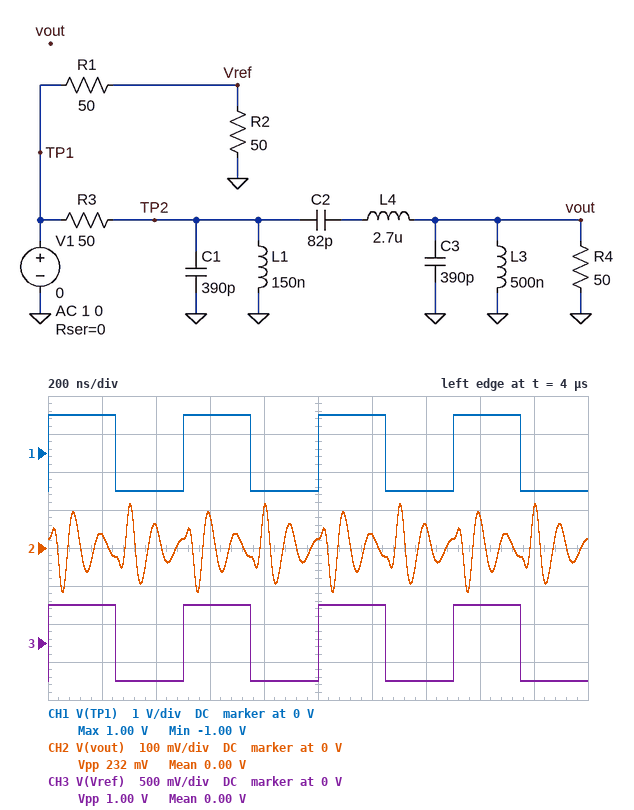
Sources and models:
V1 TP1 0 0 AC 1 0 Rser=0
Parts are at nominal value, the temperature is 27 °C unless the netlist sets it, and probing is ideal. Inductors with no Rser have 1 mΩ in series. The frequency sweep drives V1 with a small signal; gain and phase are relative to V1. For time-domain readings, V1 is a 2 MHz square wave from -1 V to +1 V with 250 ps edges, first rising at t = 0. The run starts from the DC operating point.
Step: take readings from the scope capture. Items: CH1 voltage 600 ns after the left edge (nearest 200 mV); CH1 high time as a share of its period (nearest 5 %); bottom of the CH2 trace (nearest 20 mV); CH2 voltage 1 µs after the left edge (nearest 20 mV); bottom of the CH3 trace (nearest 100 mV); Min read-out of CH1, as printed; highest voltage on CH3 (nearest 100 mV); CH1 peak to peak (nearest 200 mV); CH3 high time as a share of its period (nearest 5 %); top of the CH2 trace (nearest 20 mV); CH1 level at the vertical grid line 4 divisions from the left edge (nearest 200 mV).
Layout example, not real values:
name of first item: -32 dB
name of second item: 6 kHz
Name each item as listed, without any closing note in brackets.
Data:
CH1 voltage 600 ns after the left edge: 1.0 V
CH1 high time as a share of its period: 50 %
bottom of the CH2 trace: -120 mV
CH2 voltage 1 µs after the left edge: 20 mV
bottom of the CH3 trace: -500 mV
Min read-out of CH1, as printed: -1.00 V
highest voltage on CH3: 500 mV
CH1 peak to peak: 2.0 V
CH3 high time as a share of its period: 50 %
top of the CH2 trace: 120 mV
CH1 level at the vertical grid line 4 divisions from the left edge: -1.0 V
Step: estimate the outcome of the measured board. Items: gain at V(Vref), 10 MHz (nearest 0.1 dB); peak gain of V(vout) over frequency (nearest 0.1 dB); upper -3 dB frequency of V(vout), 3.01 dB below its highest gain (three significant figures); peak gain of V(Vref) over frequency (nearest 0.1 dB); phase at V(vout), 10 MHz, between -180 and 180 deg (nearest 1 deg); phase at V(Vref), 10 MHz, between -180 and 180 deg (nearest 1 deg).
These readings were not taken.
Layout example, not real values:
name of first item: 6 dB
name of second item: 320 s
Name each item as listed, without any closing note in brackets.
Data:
gain at V(Vref), 10 MHz: -6.0 dB
peak gain of V(vout) over frequency: -12.5 dB
upper -3 dB frequency of V(vout), 3.01 dB below its highest gain: 14.3 MHz
peak gain of V(Vref) over frequency: -6.0 dB
phase at V(vout), 10 MHz, between -180 and 180 deg: 92 deg
phase at V(Vref), 10 MHz, between -180 and 180 deg: 0 deg
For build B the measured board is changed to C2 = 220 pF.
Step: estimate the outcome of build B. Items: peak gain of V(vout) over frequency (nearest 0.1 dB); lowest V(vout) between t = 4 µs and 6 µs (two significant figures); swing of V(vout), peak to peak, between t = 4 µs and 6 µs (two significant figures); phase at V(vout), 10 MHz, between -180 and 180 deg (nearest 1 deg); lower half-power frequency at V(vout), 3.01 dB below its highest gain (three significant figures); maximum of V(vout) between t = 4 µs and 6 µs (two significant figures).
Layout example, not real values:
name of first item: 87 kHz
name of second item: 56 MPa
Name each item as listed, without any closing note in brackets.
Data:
peak gain of V(vout) over frequency: -12.1 dB
lowest V(vout) between t = 4 µs and 6 µs: -130 mV
swing of V(vout), peak to peak, between t = 4 µs and 6 µs: 260 mV
phase at V(vout), 10 MHz, between -180 and 180 deg: 27 deg
lower half-power frequency at V(vout), 3.01 dB below its highest gain: 5.60 MHz
maximum of V(vout) between t = 4 µs and 6 µs: 130 mV
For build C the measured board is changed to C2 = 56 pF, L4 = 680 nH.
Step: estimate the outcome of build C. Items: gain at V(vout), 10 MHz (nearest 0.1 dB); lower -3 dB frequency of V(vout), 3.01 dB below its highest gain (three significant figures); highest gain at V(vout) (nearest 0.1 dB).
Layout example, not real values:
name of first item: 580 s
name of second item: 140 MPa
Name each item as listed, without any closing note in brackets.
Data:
gain at V(vout), 10 MHz: -25.8 dB
lower -3 dB frequency of V(vout), 3.01 dB below its highest gain: 28.2 MHz
highest gain at V(vout): -6.8 dB
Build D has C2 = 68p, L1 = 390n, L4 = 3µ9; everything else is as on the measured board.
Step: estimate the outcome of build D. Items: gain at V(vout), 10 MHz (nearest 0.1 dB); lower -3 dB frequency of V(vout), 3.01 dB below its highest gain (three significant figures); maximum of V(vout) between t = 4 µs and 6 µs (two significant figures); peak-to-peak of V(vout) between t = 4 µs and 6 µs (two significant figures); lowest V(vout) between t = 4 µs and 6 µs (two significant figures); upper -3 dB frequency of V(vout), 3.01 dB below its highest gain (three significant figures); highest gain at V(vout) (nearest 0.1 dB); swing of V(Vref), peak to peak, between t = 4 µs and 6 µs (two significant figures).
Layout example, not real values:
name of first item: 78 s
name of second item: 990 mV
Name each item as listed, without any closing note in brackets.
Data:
gain at V(vout), 10 MHz: -7.9 dB
lower -3 dB frequency of V(vout), 3.01 dB below its highest gain: 8.13 MHz
maximum of V(vout) between t = 4 µs and 6 µs: 150 mV
peak-to-peak of V(vout) between t = 4 µs and 6 µs: 310 mV
lowest V(vout) between t = 4 µs and 6 µs: -150 mV
upper -3 dB frequency of V(vout), 3.01 dB below its highest gain: 12.0 MHz
highest gain at V(vout): -6.3 dB
swing of V(Vref), peak to peak, between t = 4 µs and 6 µs: 1.0 V
